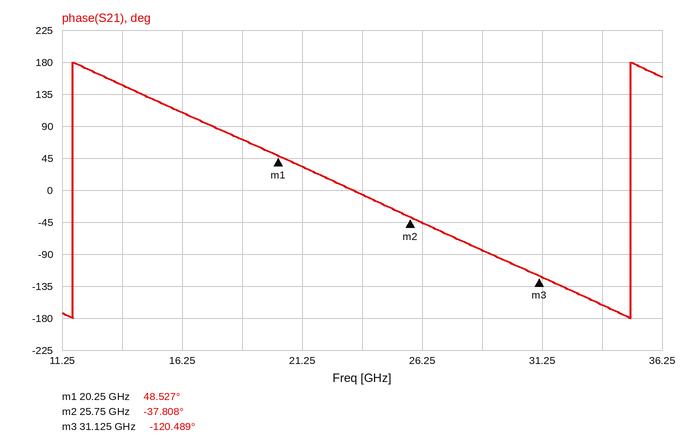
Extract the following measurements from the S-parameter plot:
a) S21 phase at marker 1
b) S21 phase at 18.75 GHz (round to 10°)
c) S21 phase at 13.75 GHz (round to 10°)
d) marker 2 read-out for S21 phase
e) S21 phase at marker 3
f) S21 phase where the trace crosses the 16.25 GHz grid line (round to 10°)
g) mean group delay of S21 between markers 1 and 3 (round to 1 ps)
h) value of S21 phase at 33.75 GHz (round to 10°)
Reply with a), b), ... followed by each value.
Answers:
a) 48.527°
b) 70°
c) 150°
d) -37.808°
e) -120.489°
f) 110°
g) 43 ps
h) -160°
